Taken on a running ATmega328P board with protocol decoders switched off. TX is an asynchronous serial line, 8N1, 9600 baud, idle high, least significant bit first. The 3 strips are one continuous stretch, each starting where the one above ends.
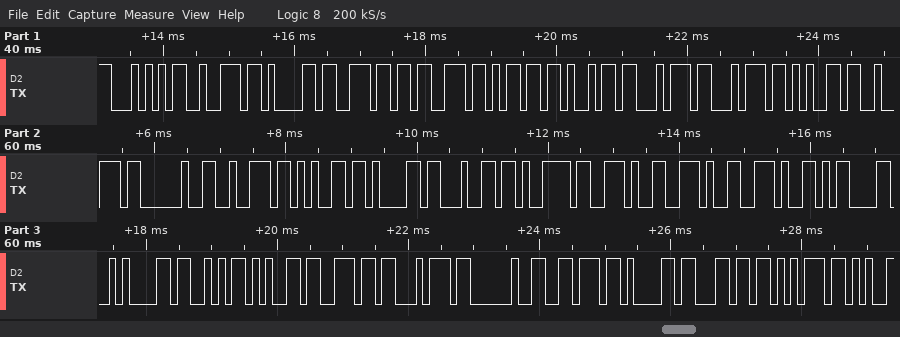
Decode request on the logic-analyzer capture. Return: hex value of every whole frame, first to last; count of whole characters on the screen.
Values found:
54 72 61 6E 73 6D 69 74 74 65 72 20 72 65 61 64 79 2E 2E 2E 0D 0A 53 65 6E 74 20 76 61 6C 75
31
